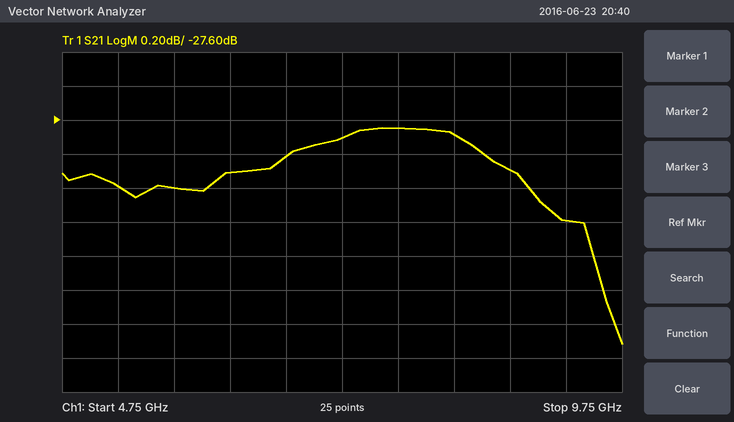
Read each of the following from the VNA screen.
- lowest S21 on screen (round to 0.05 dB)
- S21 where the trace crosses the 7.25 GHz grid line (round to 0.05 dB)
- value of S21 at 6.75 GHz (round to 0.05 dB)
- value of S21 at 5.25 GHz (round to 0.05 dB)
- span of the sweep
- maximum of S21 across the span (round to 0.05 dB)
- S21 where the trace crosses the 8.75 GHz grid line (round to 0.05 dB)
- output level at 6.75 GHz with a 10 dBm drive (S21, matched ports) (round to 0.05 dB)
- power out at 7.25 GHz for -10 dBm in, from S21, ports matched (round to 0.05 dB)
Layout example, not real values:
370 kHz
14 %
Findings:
-28.90 dB
-27.70 dB
-27.80 dB
-28.00 dB
5 GHz
-27.65 dB
-27.90 dB
-17.80 dBm
-37.70 dBm
